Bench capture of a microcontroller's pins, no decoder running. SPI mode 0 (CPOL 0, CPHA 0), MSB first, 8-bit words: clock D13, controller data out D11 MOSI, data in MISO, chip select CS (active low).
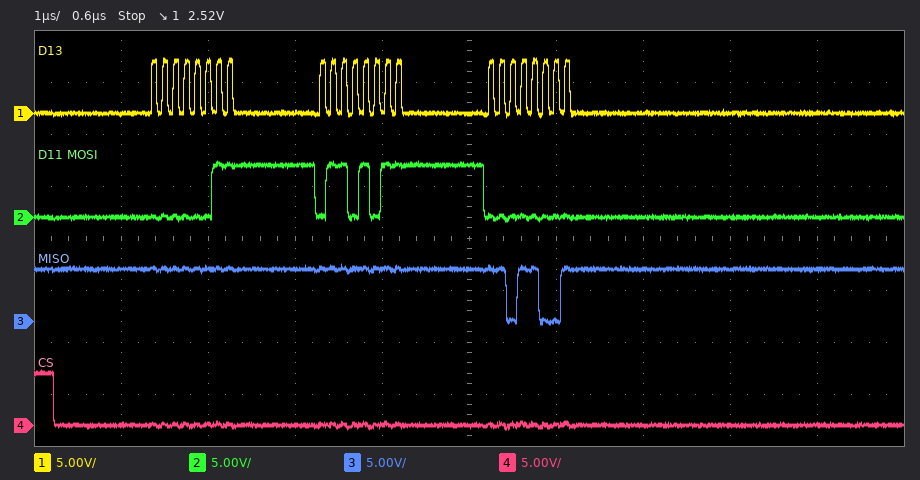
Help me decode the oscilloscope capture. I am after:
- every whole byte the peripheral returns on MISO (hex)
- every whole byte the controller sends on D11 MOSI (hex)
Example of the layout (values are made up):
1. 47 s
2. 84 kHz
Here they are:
1. FF FF D9
2. 03 6B 00
